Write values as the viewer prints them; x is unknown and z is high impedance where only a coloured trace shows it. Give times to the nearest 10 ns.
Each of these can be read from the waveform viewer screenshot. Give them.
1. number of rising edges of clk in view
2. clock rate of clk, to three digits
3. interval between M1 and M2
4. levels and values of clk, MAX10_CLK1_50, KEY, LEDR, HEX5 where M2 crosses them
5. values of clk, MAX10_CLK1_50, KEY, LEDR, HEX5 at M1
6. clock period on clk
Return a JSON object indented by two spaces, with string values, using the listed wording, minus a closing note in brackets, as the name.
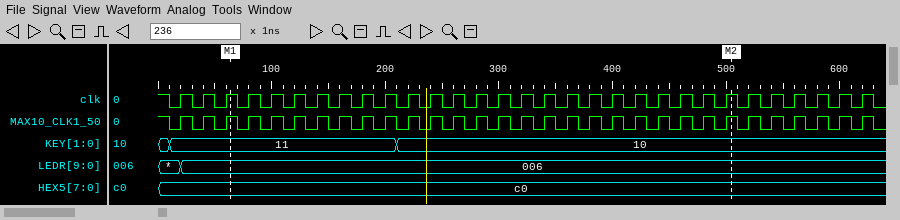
{
  "number of rising edges of clk in view": "31",
  "clock rate of clk, to three digits": "50.0 MHz",
  "interval between M1 and M2": "440 ns",
  "levels and values of clk, MAX10_CLK1_50, KEY, LEDR, HEX5 where M2 crosses them": "clk=1, MAX10_CLK1_50=1, KEY=10, LEDR=006, HEX5=c0",
  "values of clk, MAX10_CLK1_50, KEY, LEDR, HEX5 at M1": "clk=1, MAX10_CLK1_50=1, KEY=11, LEDR=006, HEX5=c0",
  "clock period on clk": "20 ns"
}
